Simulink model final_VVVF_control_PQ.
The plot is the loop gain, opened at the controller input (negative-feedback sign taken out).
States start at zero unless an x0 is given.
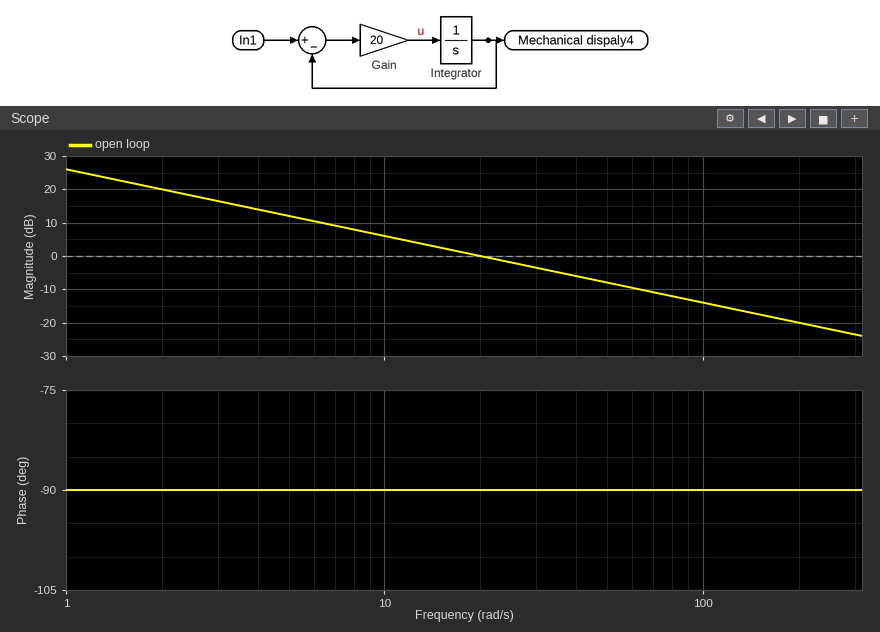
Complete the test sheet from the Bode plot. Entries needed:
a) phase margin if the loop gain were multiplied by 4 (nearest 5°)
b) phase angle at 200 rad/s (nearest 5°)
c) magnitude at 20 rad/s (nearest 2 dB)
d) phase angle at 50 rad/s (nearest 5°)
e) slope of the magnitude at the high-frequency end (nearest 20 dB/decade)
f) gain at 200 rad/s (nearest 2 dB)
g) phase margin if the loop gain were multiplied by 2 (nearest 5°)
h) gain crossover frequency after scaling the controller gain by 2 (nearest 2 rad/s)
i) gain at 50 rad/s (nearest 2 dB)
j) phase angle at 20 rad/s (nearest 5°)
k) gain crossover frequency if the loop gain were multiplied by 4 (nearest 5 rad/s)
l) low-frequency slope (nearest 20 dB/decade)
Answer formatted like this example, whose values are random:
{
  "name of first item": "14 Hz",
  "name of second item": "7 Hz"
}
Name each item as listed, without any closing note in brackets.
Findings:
{
  "phase margin if the loop gain were multiplied by 4": "90°",
  "phase angle at 200 rad/s": "-90°",
  "magnitude at 20 rad/s": "0 dB",
  "phase angle at 50 rad/s": "-90°",
  "slope of the magnitude at the high-frequency end": "-20 dB/decade",
  "gain at 200 rad/s": "-20 dB",
  "phase margin if the loop gain were multiplied by 2": "90°",
  "gain crossover frequency after scaling the controller gain by 2": "40 rad/s",
  "gain at 50 rad/s": "-8 dB",
  "phase angle at 20 rad/s": "-90°",
  "gain crossover frequency if the loop gain were multiplied by 4": "80 rad/s",
  "low-frequency slope": "-20 dB/decade"
}
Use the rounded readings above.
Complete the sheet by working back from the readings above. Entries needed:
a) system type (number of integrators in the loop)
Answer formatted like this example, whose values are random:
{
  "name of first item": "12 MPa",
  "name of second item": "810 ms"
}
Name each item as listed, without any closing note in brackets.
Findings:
{
  "system type": "1"
}
